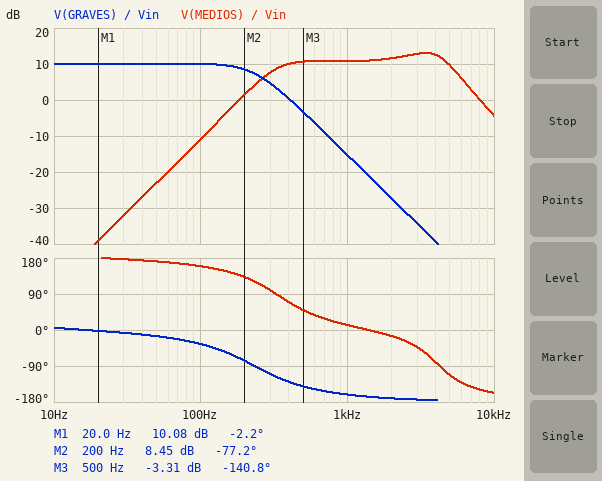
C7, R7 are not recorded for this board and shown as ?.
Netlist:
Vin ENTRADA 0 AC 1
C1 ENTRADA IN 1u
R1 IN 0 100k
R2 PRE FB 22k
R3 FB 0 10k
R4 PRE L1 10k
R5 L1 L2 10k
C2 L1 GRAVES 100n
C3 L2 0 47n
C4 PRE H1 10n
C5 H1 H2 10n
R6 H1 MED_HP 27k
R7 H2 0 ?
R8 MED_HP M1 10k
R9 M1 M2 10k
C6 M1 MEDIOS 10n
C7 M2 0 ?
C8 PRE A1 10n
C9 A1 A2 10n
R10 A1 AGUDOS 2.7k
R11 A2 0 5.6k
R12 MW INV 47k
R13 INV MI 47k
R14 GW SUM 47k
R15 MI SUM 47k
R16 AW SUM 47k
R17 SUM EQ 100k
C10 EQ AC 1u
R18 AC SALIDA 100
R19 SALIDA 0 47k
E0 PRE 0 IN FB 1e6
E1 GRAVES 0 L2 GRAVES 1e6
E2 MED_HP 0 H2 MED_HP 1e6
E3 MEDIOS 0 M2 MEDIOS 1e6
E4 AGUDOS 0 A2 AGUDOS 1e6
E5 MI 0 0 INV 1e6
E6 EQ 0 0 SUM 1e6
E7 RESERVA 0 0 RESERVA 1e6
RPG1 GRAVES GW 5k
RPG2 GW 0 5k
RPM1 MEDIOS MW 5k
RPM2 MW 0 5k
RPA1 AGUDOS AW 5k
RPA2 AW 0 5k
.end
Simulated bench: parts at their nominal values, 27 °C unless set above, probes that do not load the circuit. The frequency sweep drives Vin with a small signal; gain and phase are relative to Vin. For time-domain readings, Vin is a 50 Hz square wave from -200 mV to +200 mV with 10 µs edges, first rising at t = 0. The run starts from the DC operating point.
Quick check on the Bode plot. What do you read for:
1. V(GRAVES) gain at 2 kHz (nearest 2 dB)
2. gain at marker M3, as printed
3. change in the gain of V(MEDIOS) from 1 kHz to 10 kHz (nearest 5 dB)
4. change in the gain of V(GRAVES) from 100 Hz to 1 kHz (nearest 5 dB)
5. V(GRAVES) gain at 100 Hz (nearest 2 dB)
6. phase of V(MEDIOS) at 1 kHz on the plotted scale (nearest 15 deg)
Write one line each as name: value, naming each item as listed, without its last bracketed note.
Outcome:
V(GRAVES) gain at 2 kHz: -28 dB
gain at marker M3, as printed: -3.31 dB
change in the gain of V(MEDIOS) from 1 kHz to 10 kHz: -15 dB
change in the gain of V(GRAVES) from 100 Hz to 1 kHz: -25 dB
V(GRAVES) gain at 100 Hz: 10 dB
phase of V(MEDIOS) at 1 kHz on the plotted scale: 15 deg
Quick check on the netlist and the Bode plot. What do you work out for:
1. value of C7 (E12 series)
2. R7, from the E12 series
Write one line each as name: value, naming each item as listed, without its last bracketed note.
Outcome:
value of C7: 1.5 nF
R7, from the E12 series: 82 kΩ
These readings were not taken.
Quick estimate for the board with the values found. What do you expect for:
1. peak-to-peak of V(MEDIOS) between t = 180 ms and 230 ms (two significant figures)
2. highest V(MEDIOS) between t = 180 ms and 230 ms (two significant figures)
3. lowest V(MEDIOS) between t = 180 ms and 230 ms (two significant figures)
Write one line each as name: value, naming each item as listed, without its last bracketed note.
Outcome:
peak-to-peak of V(MEDIOS) between t = 180 ms and 230 ms: 2.7 V
highest V(MEDIOS) between t = 180 ms and 230 ms: 1.4 V
lowest V(MEDIOS) between t = 180 ms and 230 ms: -1.4 V
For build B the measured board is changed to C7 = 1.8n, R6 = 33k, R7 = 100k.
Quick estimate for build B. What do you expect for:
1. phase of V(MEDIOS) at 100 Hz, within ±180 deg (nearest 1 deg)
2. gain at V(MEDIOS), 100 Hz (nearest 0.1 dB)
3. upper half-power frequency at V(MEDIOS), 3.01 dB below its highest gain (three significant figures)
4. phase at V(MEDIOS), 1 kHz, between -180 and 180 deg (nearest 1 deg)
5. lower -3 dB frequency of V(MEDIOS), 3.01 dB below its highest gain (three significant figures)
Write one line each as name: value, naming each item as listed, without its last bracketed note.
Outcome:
phase of V(MEDIOS) at 100 Hz, within ±180 deg: 154 deg
gain at V(MEDIOS), 100 Hz: -7.3 dB
upper half-power frequency at V(MEDIOS), 3.01 dB below its highest gain: 4.45 kHz
phase at V(MEDIOS), 1 kHz, between -180 and 180 deg: 5 deg
lower -3 dB frequency of V(MEDIOS), 3.01 dB below its highest gain: 294 Hz
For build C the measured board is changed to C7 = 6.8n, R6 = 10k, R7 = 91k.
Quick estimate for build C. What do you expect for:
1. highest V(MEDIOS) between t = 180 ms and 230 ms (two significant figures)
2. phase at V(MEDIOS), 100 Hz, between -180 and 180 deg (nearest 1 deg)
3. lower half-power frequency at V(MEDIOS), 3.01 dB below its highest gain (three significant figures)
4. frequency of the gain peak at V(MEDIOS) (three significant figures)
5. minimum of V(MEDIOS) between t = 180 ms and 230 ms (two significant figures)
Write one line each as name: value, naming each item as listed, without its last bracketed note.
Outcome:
highest V(MEDIOS) between t = 180 ms and 230 ms: 780 mV
phase at V(MEDIOS), 100 Hz, between -180 and 180 deg: 169 deg
lower half-power frequency at V(MEDIOS), 3.01 dB below its highest gain: 442 Hz
frequency of the gain peak at V(MEDIOS): 590 Hz
minimum of V(MEDIOS) between t = 180 ms and 230 ms: -780 mV
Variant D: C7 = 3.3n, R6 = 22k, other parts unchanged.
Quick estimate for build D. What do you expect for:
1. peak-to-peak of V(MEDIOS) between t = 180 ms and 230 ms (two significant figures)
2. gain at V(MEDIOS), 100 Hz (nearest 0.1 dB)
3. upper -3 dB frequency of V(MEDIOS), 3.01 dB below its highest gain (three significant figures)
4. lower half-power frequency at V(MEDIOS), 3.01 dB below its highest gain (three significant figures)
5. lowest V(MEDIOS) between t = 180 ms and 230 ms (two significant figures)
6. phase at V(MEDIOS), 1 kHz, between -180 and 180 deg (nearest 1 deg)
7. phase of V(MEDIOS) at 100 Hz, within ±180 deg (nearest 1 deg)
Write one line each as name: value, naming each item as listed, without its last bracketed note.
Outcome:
peak-to-peak of V(MEDIOS) between t = 180 ms and 230 ms: 2.1 V
gain at V(MEDIOS), 100 Hz: -12.6 dB
upper -3 dB frequency of V(MEDIOS), 3.01 dB below its highest gain: 2.98 kHz
lower half-power frequency at V(MEDIOS), 3.01 dB below its highest gain: 324 Hz
lowest V(MEDIOS) between t = 180 ms and 230 ms: -1.1 V
phase at V(MEDIOS), 1 kHz, between -180 and 180 deg: -1 deg
phase of V(MEDIOS) at 100 Hz, within ±180 deg: 162 deg
